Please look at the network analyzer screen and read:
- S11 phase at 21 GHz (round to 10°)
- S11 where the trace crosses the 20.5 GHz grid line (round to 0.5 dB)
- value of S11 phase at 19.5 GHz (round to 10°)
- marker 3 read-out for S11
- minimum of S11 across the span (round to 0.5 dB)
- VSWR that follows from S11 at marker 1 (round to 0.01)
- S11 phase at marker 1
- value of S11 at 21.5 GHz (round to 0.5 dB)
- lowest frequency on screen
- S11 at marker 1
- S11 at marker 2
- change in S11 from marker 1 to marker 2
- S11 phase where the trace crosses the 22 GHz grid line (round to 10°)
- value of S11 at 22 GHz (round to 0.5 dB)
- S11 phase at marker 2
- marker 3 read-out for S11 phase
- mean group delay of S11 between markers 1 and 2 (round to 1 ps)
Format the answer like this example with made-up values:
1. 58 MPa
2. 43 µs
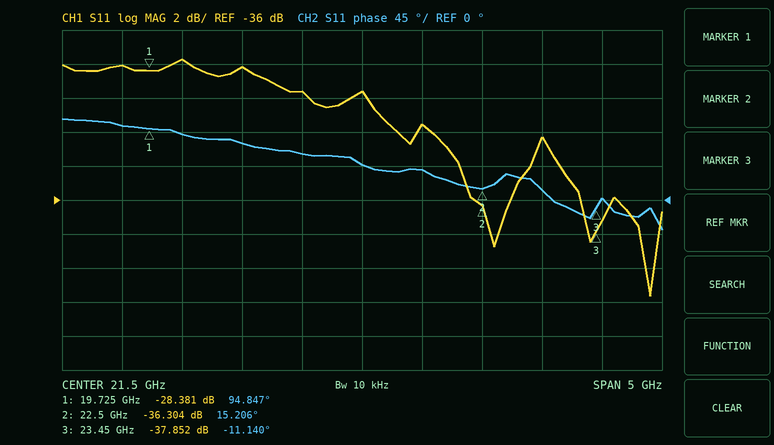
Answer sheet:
1. 60°
2. -28.0 dB
3. 100°
4. -37.852 dB
5. -41.5 dB
6. 1.08
7. 94.847°
8. -29.5 dB
9. 19 GHz
10. -28.381 dB
11. -36.304 dB
12. -7.923 dB
13. 40°
14. -31.5 dB
15. 15.206°
16. -11.140°
17. 80 ps
